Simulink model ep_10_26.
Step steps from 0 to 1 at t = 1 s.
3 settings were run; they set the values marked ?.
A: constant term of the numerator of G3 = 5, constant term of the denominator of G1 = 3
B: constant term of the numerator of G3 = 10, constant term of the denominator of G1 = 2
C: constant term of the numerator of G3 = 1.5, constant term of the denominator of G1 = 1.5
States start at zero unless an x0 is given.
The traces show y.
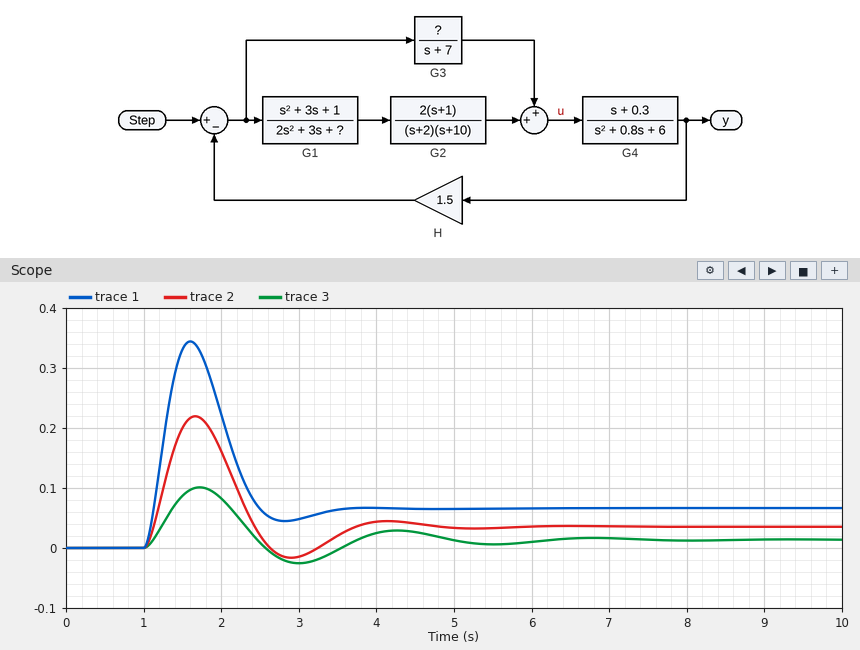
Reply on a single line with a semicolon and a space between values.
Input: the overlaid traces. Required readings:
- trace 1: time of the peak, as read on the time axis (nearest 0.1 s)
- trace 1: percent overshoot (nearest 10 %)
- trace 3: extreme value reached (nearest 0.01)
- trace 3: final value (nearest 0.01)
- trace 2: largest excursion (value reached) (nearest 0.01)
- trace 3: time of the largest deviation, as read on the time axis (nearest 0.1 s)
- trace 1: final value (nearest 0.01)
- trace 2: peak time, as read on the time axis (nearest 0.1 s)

1.6 s; 420 %; 0.10; 0.01; 0.22; 1.7 s; 0.07; 1.7 s
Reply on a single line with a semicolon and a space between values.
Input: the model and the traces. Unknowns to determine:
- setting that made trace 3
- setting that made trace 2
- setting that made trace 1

C; A; B
